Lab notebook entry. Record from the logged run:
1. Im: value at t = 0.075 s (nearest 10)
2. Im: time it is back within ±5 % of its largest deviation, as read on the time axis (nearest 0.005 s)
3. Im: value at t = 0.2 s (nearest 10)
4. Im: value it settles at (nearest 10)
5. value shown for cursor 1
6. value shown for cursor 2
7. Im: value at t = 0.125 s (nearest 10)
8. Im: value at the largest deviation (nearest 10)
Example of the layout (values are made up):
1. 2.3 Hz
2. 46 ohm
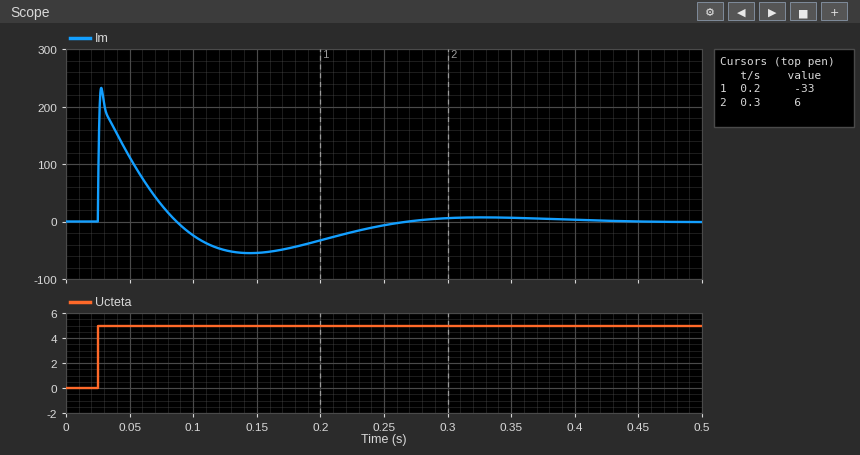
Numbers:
1. 30
2. 0.240 s
3. -30
4. 0
5. -33
6. 6
7. -50
8. 230
